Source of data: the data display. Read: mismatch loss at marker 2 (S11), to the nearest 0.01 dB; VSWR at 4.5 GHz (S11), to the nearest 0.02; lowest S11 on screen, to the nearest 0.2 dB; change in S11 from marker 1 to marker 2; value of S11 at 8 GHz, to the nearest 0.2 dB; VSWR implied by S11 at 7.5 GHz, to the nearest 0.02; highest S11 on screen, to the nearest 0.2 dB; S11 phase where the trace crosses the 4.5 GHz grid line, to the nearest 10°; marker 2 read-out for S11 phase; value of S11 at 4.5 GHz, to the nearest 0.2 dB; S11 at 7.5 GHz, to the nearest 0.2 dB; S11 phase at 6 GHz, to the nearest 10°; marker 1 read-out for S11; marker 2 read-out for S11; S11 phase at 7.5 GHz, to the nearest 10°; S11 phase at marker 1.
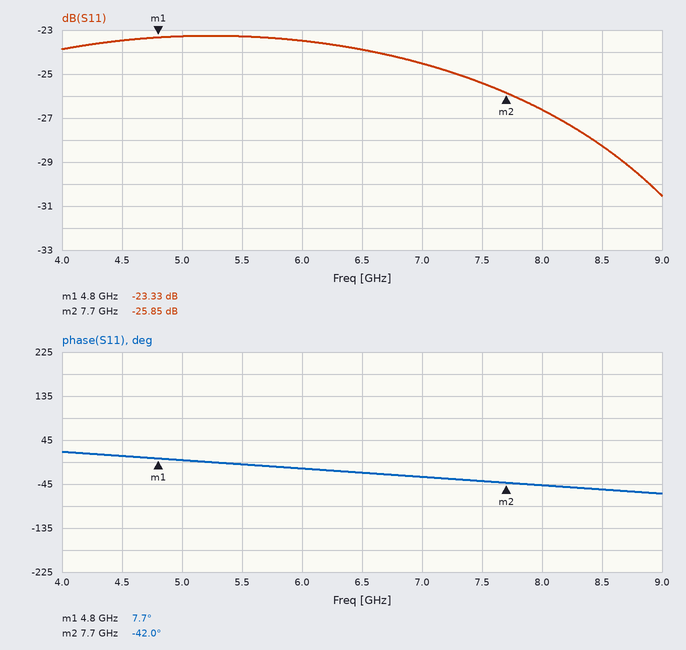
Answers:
0.01 dB
1.14
-30.6 dB
-2.52 dB
-26.6 dB
1.12
-23.2 dB
10°
-42.0°
-23.4 dB
-25.4 dB
-10°
-23.33 dB
-25.85 dB
-40°
7.7°
